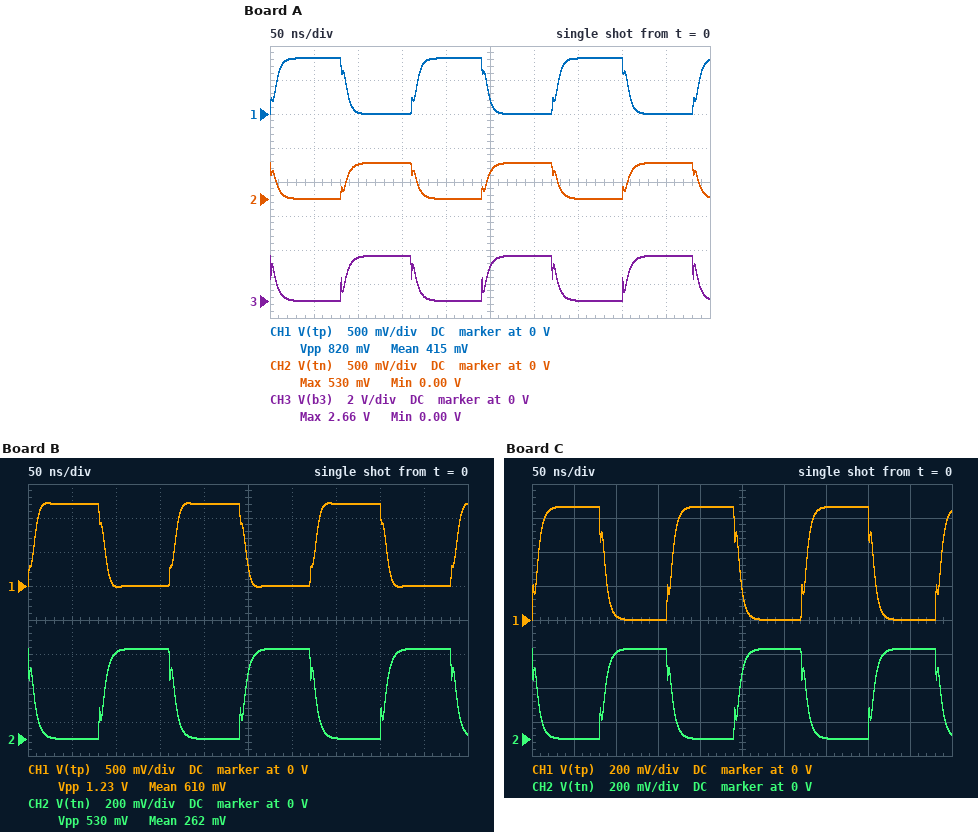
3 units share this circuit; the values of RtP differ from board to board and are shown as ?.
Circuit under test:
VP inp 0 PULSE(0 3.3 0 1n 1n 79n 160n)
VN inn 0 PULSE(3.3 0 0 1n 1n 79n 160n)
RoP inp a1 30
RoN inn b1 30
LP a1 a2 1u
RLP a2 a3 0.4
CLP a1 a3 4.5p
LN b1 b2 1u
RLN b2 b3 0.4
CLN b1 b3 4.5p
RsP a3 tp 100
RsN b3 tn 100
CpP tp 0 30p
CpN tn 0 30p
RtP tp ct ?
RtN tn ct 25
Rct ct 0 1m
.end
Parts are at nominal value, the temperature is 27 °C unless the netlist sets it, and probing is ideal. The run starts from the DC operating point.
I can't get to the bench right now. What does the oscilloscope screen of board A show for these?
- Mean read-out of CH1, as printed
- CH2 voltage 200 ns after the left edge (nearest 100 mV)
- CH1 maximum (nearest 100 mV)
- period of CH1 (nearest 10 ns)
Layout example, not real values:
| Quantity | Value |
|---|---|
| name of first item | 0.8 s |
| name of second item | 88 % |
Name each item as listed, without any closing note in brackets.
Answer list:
| Quantity | Value |
|---|---|
| Mean read-out of CH1, as printed | 415 mV |
| CH2 voltage 200 ns after the left edge | 0 V |
| CH1 maximum | 800 mV |
| period of CH1 | 160 ns |
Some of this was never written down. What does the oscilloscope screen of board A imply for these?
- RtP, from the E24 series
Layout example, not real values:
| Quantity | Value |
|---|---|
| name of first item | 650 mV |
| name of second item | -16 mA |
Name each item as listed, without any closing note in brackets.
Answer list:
| Quantity | Value |
|---|---|
| RtP, from the E24 series | 43 Ω |
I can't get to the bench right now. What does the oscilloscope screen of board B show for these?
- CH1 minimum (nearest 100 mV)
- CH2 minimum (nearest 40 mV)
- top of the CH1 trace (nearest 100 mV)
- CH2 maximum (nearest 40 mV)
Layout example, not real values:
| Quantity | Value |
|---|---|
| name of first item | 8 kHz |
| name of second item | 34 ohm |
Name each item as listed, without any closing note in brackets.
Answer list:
| Quantity | Value |
|---|---|
| CH1 minimum | 0 V |
| CH2 minimum | 0 V |
| top of the CH1 trace | 1.2 V |
| CH2 maximum | 520 mV |
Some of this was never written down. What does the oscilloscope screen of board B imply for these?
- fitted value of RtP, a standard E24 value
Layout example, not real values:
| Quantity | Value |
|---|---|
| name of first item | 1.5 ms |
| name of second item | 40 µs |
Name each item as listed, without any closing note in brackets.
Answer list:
| Quantity | Value |
|---|---|
| fitted value of RtP, a standard E24 value | 75 Ω |
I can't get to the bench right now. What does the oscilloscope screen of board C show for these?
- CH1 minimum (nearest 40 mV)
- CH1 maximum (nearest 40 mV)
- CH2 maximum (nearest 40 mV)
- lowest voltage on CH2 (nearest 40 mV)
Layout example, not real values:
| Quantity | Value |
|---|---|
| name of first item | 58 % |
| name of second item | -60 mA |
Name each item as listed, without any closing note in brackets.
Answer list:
| Quantity | Value |
|---|---|
| CH1 minimum | 0 V |
| CH1 maximum | 680 mV |
| CH2 maximum | 520 mV |
| lowest voltage on CH2 | 0 V |
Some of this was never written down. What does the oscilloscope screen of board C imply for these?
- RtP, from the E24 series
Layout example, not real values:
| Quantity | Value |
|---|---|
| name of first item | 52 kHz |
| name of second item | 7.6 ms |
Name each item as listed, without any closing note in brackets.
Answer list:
| Quantity | Value |
|---|---|
| RtP, from the E24 series | 33 Ω |
